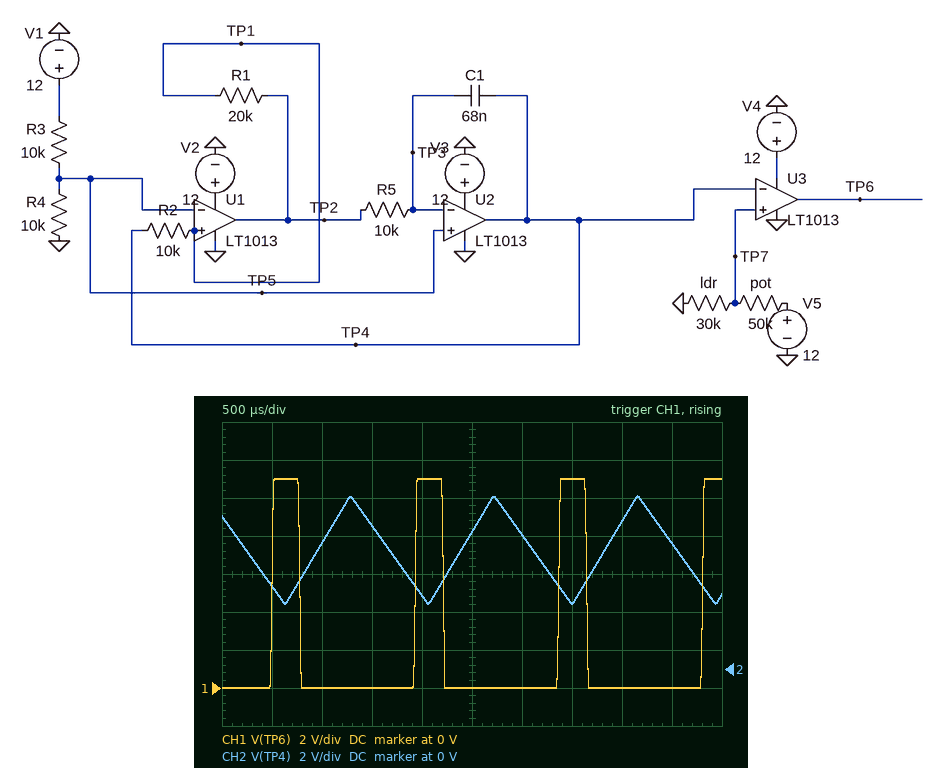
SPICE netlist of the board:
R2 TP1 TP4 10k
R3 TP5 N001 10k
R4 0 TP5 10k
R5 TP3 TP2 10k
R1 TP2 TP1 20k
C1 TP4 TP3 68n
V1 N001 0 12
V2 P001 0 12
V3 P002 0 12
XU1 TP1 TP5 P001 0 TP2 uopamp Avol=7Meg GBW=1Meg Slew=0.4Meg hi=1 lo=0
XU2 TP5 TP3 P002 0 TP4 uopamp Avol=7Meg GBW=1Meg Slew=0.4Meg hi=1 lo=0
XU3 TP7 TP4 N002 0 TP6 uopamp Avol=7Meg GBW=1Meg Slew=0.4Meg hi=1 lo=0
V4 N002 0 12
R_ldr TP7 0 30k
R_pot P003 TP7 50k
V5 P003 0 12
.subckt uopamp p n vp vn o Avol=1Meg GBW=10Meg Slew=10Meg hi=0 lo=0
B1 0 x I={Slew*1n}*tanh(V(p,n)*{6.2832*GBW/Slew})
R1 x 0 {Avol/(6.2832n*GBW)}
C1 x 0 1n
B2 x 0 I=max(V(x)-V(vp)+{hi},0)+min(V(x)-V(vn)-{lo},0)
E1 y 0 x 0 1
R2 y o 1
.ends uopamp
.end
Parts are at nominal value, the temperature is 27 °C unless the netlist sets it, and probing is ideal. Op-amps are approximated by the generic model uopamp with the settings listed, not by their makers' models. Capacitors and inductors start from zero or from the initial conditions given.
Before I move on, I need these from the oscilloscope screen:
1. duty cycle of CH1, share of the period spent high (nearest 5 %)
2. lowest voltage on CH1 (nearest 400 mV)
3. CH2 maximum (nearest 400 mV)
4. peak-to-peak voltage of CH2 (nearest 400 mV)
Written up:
20 %
0 V
9.2 V
5.6 V
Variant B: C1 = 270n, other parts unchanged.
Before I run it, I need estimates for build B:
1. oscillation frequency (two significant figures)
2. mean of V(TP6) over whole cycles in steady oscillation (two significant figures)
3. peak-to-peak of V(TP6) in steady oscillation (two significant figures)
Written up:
180 Hz
2.0 V
11 V
